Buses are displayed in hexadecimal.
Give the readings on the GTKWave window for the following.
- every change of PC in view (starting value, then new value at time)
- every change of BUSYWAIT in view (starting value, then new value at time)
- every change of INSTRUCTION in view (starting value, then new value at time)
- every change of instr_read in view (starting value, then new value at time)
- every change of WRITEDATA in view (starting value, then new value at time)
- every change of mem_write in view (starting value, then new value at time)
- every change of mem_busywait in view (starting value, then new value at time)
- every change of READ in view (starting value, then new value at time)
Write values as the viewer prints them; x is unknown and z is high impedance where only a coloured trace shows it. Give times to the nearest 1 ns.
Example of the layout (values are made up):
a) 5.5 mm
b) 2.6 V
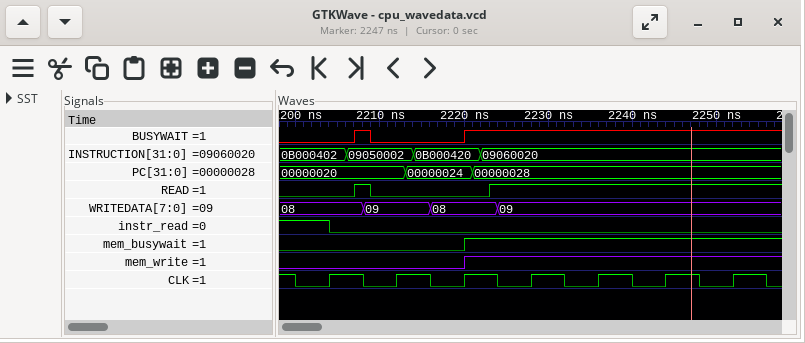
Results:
a) 00000020, 00000024 at 2213 ns, 00000028 at 2221 ns
b) 0, 1 at 2207 ns, 0 at 2209 ns, 1 at 2220 ns
c) 0B000402, 09050002 at 2206 ns, 0B000420 at 2214 ns, 09060020 at 2222 ns
d) 1, 0 at 2204 ns
e) 08, 09 at 2208 ns, 08 at 2216 ns, 09 at 2224 ns
f) 0, 1 at 2220 ns
g) 0, 1 at 2220 ns
h) 0, 1 at 2207 ns, 0 at 2209 ns, 1 at 2223 ns
